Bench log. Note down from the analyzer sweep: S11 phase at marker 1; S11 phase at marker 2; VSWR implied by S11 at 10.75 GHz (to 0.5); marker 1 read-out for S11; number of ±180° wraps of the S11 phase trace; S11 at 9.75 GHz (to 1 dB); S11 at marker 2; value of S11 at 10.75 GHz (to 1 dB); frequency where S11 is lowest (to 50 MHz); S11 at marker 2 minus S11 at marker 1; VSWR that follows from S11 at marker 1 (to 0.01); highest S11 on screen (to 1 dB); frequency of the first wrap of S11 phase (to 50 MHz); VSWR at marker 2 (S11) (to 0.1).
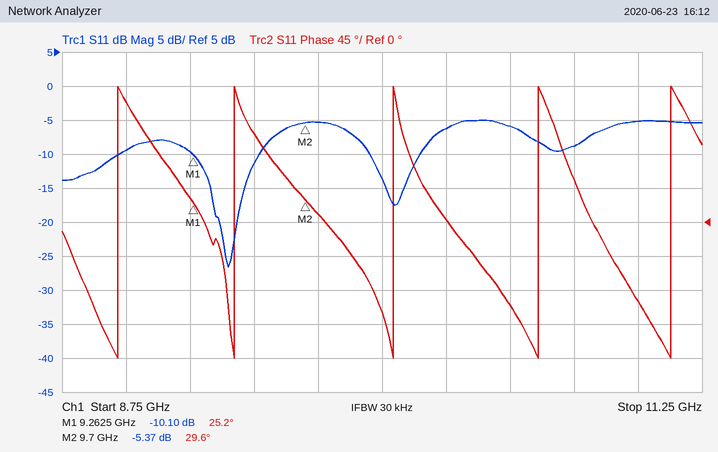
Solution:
25.2°
29.6°
2.0
-10.10 dB
5
-5 dB
-5.37 dB
-9 dB
9.40 GHz
4.73 dB
1.91
-5 dB
8.95 GHz
3.3
